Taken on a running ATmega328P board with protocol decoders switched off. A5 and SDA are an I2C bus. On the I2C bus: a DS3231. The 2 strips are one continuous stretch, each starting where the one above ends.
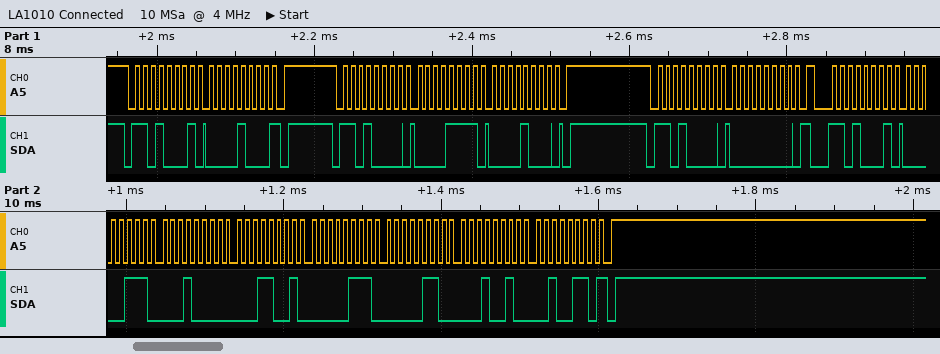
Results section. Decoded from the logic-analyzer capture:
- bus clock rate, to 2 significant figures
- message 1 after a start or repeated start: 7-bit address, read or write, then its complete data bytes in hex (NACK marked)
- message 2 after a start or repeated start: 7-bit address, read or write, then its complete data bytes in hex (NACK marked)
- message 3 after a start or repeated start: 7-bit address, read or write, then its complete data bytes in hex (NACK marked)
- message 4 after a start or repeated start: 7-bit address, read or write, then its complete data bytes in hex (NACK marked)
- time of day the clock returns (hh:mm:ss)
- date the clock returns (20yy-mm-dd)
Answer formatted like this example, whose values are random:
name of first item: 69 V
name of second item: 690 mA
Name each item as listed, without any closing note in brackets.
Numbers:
bus clock rate, to 2 significant figures: 100 kHz
message 1 after a start or repeated start: 7-bit address, read or write, then its complete data bytes in hex: 0x68 read: 08 NACK
message 2 after a start or repeated start: 7-bit address, read or write, then its complete data bytes in hex: 0x68 write: 0F 08
message 3 after a start or repeated start: 7-bit address, read or write, then its complete data bytes in hex: 0x68 write: 00
message 4 after a start or repeated start: 7-bit address, read or write, then its complete data bytes in hex: 0x68 read: 07 10 19 07 06 12 26 NACK
time of day the clock returns: 19:10:07
date the clock returns: 2026-12-06
